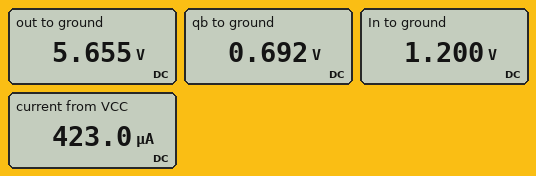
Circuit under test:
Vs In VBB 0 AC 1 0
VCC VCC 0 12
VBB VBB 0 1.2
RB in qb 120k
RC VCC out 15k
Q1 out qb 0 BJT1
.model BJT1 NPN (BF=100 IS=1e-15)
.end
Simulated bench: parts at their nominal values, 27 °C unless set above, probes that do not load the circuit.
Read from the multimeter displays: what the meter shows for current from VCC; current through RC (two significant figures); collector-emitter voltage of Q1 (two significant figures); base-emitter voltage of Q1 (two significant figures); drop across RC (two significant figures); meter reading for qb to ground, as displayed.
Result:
423.0 µA
420 µA
5.7 V
690 mV
6.3 V
0.692 V
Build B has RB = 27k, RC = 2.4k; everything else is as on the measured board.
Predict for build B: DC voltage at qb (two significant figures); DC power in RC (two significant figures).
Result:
730 mV
7.3 mW
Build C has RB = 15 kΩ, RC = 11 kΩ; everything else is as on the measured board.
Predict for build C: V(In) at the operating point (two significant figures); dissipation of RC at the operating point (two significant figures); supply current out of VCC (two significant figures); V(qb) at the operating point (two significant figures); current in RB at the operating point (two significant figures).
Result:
1.2 V
13 mW
1.1 mA
720 mV
32 µA
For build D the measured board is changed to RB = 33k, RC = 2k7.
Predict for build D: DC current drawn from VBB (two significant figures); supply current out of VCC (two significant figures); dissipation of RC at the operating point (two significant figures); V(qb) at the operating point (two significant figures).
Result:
14 µA
1.4 mA
5.6 mW
720 mV
